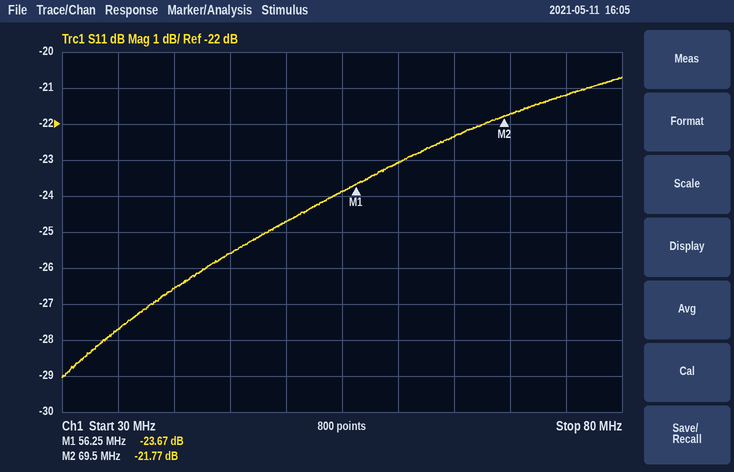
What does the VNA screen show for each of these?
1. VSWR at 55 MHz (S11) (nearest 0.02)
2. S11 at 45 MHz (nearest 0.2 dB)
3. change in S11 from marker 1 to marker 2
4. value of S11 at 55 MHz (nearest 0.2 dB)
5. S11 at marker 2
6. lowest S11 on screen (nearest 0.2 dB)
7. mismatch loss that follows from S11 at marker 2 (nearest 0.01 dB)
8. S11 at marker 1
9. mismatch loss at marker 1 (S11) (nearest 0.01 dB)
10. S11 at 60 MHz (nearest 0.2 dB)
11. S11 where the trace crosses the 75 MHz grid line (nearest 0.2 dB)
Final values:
1.14
-25.6 dB
1.90 dB
-23.8 dB
-21.77 dB
-29.0 dB
0.03 dB
-23.67 dB
0.02 dB
-23.0 dB
-21.2 dB
